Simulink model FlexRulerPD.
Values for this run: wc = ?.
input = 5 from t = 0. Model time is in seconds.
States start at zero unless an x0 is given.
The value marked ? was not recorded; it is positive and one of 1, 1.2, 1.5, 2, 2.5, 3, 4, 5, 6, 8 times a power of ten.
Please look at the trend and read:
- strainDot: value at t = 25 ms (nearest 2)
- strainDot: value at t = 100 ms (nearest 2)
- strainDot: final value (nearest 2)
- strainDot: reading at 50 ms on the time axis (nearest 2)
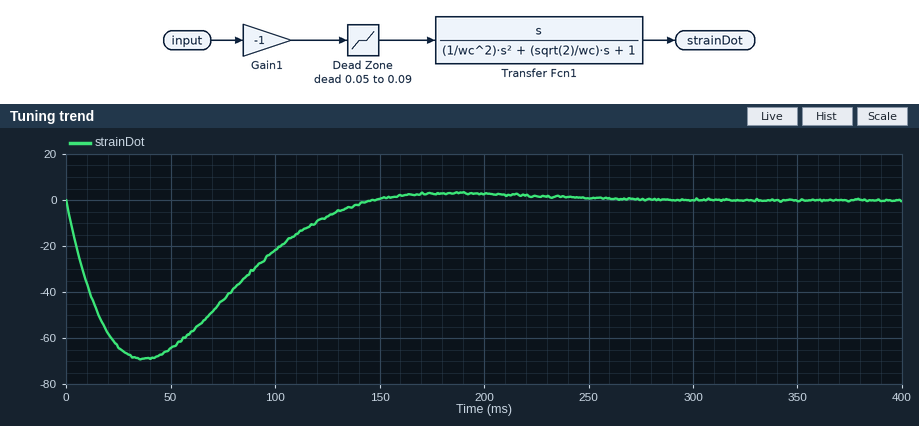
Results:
-64
-22
0
-64
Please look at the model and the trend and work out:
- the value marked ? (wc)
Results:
30
